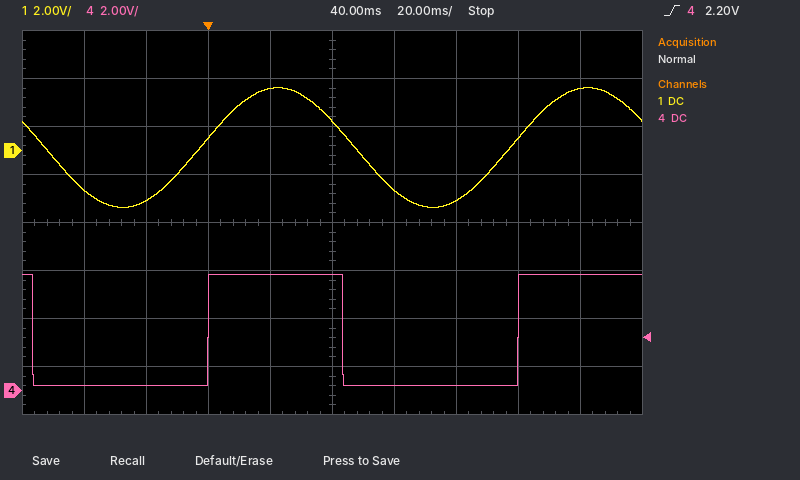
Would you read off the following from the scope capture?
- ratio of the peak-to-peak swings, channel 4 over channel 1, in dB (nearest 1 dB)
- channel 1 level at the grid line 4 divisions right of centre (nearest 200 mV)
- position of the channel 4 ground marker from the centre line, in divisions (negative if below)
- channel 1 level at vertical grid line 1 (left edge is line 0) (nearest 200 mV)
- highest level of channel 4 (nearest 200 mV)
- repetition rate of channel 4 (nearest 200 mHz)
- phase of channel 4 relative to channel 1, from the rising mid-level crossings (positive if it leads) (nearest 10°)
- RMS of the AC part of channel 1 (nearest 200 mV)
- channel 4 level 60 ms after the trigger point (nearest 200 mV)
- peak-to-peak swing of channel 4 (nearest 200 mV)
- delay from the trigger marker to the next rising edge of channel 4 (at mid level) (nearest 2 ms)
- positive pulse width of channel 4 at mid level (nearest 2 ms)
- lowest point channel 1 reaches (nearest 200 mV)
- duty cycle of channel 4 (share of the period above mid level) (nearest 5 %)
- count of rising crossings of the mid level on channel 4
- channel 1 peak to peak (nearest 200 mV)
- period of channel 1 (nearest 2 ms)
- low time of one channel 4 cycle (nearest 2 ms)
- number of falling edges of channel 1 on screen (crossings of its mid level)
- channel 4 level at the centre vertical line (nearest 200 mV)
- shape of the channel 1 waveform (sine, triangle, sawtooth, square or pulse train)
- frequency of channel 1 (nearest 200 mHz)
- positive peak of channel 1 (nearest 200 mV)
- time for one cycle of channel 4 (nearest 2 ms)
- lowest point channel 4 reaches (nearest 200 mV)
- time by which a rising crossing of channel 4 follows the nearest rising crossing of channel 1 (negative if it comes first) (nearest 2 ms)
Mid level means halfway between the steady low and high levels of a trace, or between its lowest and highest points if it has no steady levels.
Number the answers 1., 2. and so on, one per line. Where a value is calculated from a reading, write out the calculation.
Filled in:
1. 20 log10(4.6 V / 5.0 V) ≈ -1 dB
2. 2.6 V
3. -3.5 div
4. -1.6 V
5. 4.8 V
6. 1 / 100 ms ≈ 10.0 Hz
7. −360° × (+2 ms) / 100 ms ≈ -7.20°, so -10° to the nearest 10°
8. 5.0 V / (2√2) ≈ 1.8 V
9. 200 mV
10. 4.8 V − (200 mV) = 4.6 V
11. 100 ms
12. 44 ms
13. -2.4 V
14. 44 ms / 100 ms ≈ 44.0 %, so 45 % to the nearest 5 %
15. 2
16. 2.6 V − (-2.4 V) = 5.0 V
17. 100 ms
18. 56 ms
19. 2
20. 4.8 V
21. sine
22. 1 / 100 ms ≈ 10.0 Hz
23. 2.6 V
24. 100 ms
25. 200 mV
26. +2 ms
